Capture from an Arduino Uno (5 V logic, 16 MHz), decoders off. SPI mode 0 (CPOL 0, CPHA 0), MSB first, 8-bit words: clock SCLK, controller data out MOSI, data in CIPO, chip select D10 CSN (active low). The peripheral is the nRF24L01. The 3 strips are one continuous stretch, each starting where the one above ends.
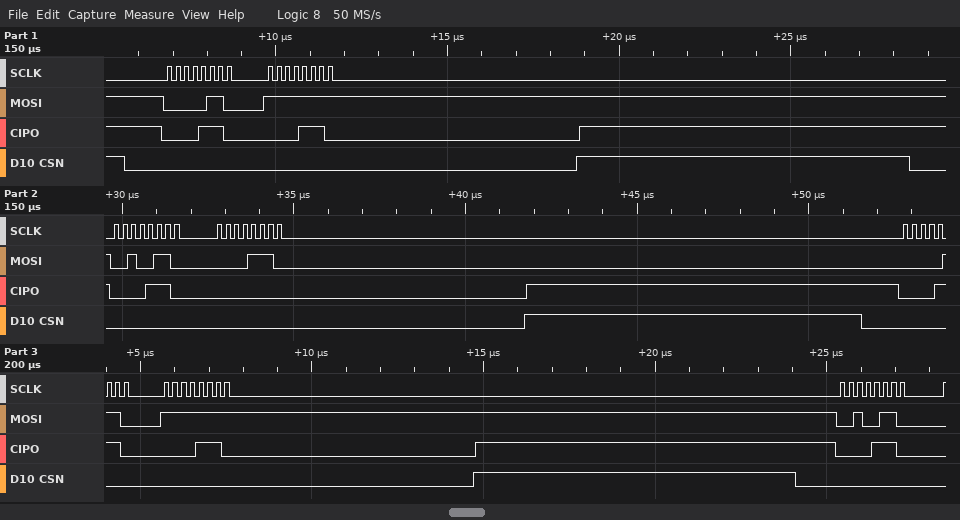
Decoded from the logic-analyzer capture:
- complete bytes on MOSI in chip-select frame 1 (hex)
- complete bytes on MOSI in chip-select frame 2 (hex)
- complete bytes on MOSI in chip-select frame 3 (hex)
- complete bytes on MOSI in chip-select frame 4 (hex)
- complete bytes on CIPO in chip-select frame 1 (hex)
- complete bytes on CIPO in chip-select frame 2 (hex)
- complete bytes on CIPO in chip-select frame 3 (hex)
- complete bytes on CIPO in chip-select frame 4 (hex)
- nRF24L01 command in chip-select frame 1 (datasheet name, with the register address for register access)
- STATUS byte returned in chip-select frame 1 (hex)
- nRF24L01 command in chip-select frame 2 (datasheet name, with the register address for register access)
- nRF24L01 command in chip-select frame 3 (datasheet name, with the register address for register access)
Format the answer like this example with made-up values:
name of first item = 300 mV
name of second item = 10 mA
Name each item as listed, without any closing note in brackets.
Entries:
complete bytes on MOSI in chip-select frame 1 = 0x06 0xFF
complete bytes on MOSI in chip-select frame 2 = 0x26 0x0E
complete bytes on MOSI in chip-select frame 3 = 0x06 0xFF
complete bytes on MOSI in chip-select frame 4 = 0x26
complete bytes on CIPO in chip-select frame 1 = 0x0E 0x0E
complete bytes on CIPO in chip-select frame 2 = 0x0E 0x00
complete bytes on CIPO in chip-select frame 3 = 0x0E 0x0E
complete bytes on CIPO in chip-select frame 4 = 0x0E
nRF24L01 command in chip-select frame 1 = R_REGISTER 0x06
STATUS byte returned in chip-select frame 1 = 0x0E
nRF24L01 command in chip-select frame 2 = W_REGISTER 0x06
nRF24L01 command in chip-select frame 3 = R_REGISTER 0x06
